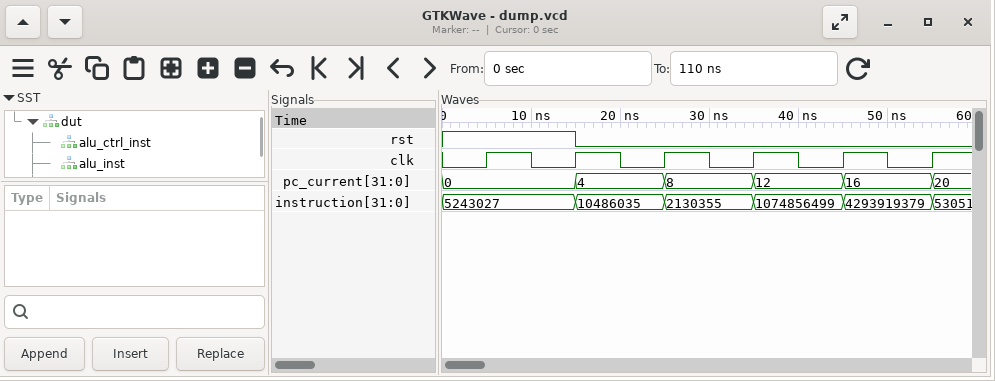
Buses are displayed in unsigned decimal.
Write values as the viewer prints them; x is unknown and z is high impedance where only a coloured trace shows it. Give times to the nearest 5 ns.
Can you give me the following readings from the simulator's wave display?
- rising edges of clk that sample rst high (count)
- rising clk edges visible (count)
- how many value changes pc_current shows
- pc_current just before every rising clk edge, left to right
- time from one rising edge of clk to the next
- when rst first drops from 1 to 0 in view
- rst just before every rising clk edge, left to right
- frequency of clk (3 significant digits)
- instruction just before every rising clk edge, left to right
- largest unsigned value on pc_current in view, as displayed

2
6
5
0, 0, 4, 8, 12, 16
10 ns
15 ns
1 1 0 0 0 0
100 MHz
5243027, 5243027, 10486035, 2130355, 1074856499, 4293919379
20
